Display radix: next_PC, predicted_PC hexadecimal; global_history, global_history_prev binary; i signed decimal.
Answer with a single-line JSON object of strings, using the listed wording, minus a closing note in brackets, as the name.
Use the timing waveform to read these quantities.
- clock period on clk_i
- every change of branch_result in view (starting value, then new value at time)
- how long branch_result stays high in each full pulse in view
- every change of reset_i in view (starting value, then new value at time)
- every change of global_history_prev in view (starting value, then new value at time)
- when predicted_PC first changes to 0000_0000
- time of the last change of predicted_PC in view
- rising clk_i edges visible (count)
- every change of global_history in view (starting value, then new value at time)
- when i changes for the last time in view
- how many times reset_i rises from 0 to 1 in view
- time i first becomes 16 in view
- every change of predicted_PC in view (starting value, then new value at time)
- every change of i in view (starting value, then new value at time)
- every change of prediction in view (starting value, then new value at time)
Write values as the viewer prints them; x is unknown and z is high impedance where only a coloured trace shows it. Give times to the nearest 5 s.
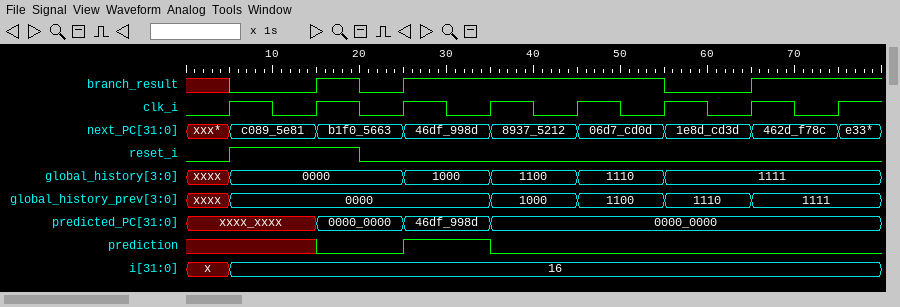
{"clock period on clk_i": "10 s", "every change of branch_result in view": "x, 0 at 5 s, 1 at 15 s, 0 at 20 s, 1 at 25 s, 0 at 55 s, 1 at 65 s", "how long branch_result stays high in each full pulse in view": "5 s, 30 s", "every change of reset_i in view": "0, 1 at 5 s, 0 at 20 s", "every change of global_history_prev in view": "xxxx, 0000 at 5 s, 1000 at 35 s, 1100 at 45 s, 1110 at 55 s, 1111 at 65 s", "when predicted_PC first changes to 0000_0000": "15 s", "time of the last change of predicted_PC in view": "35 s", "rising clk_i edges visible": "8", "every change of global_history in view": "xxxx, 0000 at 5 s, 1000 at 25 s, 1100 at 35 s, 1110 at 45 s, 1111 at 55 s", "when i changes for the last time in view": "5 s", "how many times reset_i rises from 0 to 1 in view": "1", "time i first becomes 16 in view": "5 s", "every change of predicted_PC in view": "xxxx_xxxx, 0000_0000 at 15 s, 46df_998d at 25 s, 0000_0000 at 35 s", "every change of i in view": "x, 16 at 5 s", "every change of prediction in view": "x, 0 at 15 s, 1 at 25 s, 0 at 35 s"}
